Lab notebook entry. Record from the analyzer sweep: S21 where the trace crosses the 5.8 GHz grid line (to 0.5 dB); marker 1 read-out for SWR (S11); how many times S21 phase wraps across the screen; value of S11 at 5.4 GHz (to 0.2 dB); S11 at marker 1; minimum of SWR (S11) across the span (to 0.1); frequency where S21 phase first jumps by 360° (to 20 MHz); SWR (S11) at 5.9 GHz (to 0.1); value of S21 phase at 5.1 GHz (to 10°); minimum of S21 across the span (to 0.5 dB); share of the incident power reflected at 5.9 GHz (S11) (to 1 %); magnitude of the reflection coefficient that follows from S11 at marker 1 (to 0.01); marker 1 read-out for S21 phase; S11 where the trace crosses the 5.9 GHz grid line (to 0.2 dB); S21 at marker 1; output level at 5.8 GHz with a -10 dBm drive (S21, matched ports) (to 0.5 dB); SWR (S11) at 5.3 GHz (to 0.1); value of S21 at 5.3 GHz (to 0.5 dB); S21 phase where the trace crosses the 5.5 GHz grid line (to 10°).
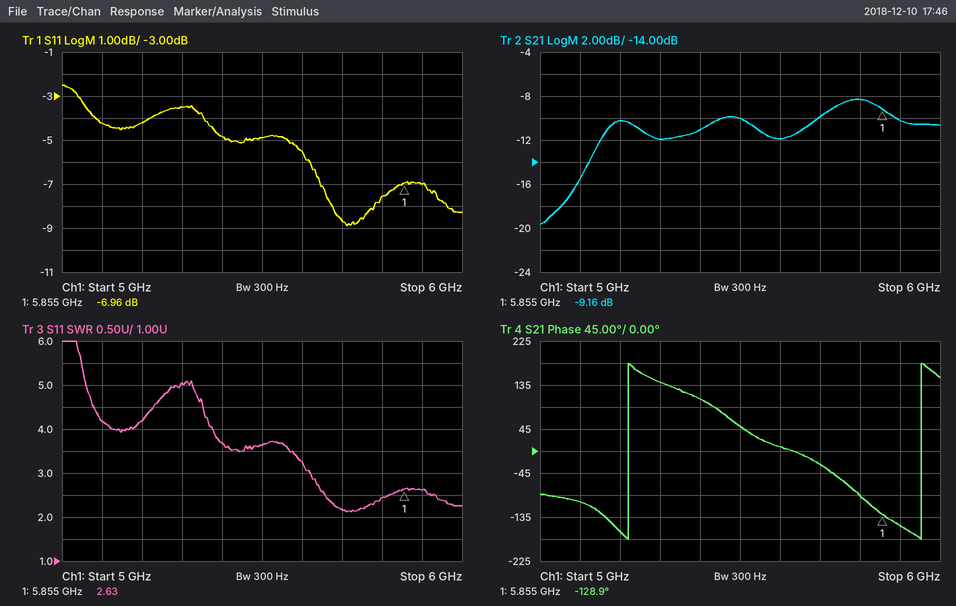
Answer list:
-8.5 dB
2.63
2
-4.8 dB
-6.96 dB
2.1
5.22 GHz
2.6
-100°
-19.5 dB
20 %
0.45
-128.9°
-7.0 dB
-9.16 dB
-18.5 dBm
5.0
-12.0 dB
50°
